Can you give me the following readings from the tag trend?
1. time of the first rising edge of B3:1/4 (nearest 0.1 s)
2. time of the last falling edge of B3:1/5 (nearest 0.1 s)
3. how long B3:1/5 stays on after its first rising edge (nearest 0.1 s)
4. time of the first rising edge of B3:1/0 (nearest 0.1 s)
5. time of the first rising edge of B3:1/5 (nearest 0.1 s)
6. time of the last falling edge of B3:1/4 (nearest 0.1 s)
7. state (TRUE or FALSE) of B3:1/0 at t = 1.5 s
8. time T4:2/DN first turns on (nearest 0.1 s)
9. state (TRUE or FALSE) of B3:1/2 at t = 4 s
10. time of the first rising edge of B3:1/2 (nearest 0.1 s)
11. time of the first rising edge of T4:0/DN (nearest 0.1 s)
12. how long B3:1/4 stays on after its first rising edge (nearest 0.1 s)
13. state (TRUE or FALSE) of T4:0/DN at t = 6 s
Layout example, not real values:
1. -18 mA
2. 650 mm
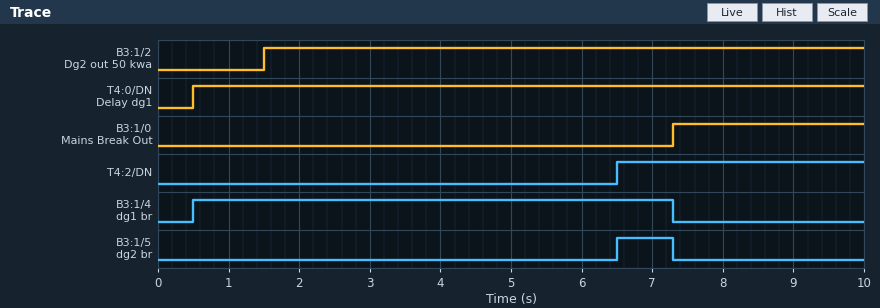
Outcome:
1. 0.5 s
2. 7.3 s
3. 0.8 s
4. 7.3 s
5. 6.5 s
6. 7.3 s
7. FALSE
8. 6.5 s
9. TRUE
10. 1.5 s
11. 0.5 s
12. 6.8 s
13. TRUE
